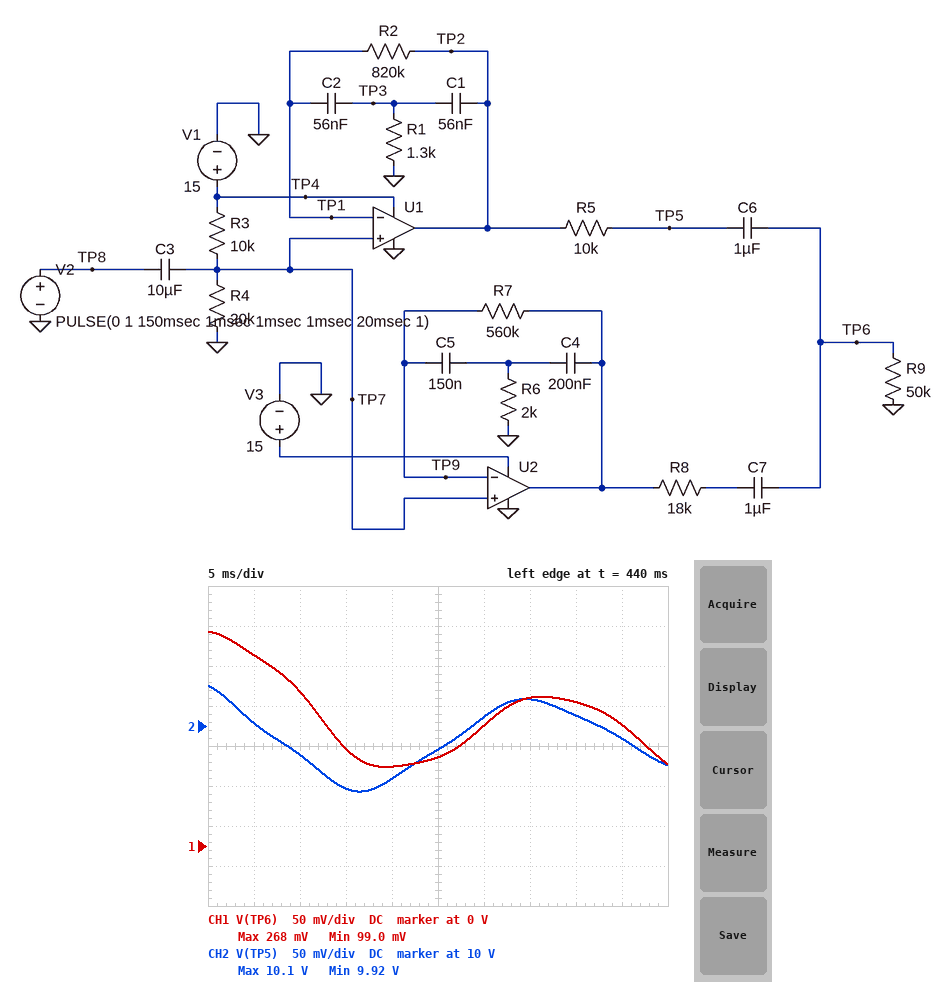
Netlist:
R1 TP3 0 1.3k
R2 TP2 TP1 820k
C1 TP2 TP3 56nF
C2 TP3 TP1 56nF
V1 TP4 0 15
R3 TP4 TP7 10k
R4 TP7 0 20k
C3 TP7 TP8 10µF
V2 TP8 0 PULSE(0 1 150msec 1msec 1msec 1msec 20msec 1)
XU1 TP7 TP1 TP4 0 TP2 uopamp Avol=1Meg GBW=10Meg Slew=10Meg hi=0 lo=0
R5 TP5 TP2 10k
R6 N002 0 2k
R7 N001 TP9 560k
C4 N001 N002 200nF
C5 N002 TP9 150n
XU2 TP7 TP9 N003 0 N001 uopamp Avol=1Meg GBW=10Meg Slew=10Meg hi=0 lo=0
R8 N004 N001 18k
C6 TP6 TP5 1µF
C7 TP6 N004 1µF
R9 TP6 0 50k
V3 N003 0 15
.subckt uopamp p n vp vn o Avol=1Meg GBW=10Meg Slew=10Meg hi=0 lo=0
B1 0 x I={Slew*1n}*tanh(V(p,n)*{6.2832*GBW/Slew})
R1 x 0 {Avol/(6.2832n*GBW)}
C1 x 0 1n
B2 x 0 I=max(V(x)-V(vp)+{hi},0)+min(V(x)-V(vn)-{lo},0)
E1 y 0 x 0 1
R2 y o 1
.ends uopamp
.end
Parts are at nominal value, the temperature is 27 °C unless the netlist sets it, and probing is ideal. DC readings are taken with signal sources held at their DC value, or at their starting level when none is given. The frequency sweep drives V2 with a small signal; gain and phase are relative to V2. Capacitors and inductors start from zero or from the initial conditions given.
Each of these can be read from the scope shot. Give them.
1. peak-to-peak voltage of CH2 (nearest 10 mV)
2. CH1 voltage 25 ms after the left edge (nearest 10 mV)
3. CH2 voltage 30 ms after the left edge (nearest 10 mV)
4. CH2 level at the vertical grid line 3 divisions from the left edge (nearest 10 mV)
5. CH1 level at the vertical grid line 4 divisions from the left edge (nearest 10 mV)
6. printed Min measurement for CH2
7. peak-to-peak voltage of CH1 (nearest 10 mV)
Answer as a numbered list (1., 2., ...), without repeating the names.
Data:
1. 130 mV
2. 110 mV
3. 10.01 V
4. 9.92 V
5. 100 mV
6. 9.92 V
7. 170 mV
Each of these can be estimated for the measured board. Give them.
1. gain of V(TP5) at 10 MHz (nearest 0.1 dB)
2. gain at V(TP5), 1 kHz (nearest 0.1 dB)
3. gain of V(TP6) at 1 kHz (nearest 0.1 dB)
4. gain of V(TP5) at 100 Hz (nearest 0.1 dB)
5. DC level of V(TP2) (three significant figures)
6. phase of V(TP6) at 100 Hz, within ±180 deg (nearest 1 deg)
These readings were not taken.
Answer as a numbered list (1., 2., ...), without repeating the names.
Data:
1. -4.1 dB
2. 4.3 dB
3. 4.3 dB
4. 34.2 dB
5. 10.0 V
6. -70 deg
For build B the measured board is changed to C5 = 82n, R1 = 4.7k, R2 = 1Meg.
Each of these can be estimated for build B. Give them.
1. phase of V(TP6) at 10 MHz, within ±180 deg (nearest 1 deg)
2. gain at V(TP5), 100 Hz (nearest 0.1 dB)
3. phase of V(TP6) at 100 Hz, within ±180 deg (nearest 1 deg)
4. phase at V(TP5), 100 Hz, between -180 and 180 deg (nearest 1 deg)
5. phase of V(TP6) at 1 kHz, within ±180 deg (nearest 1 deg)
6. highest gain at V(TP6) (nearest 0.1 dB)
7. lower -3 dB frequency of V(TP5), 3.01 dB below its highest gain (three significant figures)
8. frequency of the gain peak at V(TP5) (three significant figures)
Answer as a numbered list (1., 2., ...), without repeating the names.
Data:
1. -45 deg
2. 15.2 dB
3. -75 deg
4. -77 deg
5. -28 deg
6. 36.5 dB
7. 36.4 Hz
8. 41.4 Hz
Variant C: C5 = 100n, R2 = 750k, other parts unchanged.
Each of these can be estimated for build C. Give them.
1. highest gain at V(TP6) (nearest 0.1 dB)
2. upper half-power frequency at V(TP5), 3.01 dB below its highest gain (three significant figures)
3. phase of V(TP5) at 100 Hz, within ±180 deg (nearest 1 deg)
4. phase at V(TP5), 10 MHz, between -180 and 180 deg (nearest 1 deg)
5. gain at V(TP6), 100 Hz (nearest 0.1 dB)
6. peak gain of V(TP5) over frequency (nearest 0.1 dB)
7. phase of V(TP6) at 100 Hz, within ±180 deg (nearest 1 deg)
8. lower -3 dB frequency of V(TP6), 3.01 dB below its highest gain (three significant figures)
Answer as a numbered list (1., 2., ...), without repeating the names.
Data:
1. 44.3 dB
2. 94.9 Hz
3. -69 deg
4. -45 deg
5. 36.6 dB
6. 44.5 dB
7. -62 deg
8. 87.4 Hz
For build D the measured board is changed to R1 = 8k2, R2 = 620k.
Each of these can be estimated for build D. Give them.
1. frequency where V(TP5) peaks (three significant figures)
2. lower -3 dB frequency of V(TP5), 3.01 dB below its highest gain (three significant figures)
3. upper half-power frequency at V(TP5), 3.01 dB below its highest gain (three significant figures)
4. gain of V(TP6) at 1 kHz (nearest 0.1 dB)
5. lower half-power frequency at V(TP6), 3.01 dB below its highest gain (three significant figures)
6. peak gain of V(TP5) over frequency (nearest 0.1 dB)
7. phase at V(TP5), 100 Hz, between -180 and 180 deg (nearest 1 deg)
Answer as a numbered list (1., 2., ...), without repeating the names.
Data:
1. 27.4 Hz
2. 25.7 Hz
3. 29.1 Hz
4. -0.5 dB
5. 25.5 Hz
6. 32.4 dB
7. -71 deg
